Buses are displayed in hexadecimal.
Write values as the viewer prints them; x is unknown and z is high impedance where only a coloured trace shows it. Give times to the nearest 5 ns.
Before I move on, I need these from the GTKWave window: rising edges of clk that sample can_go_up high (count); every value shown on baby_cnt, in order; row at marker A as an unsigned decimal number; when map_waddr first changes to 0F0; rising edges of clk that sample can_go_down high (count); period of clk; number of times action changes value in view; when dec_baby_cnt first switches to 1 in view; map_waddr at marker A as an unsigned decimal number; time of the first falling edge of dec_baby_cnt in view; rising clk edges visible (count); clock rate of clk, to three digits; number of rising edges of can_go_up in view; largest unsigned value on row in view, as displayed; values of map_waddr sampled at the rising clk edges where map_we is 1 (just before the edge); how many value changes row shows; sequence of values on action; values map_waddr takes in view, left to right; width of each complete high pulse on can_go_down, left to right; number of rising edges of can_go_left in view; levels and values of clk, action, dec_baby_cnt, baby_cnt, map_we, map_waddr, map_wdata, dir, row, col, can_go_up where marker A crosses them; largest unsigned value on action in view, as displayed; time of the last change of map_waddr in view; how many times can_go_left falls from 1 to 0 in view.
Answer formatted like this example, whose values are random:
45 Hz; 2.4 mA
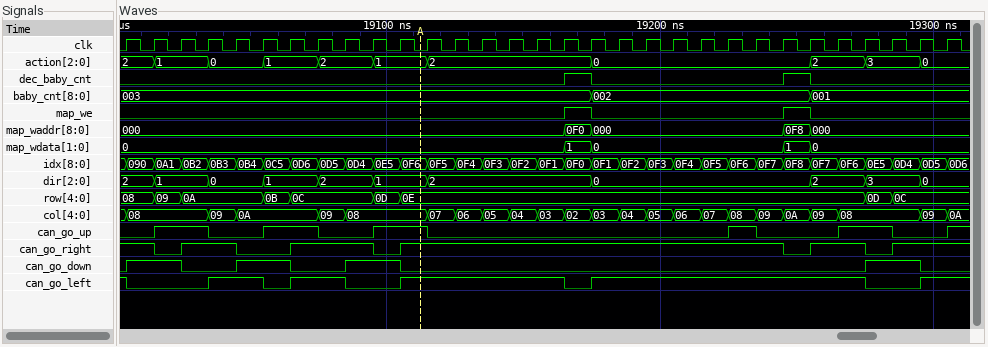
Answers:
9; 003, 002, 001; 14; 19165 ns; 8; 10 ns; 10; 19165 ns; 0; 19175 ns; 31; 100 MHz; 6; 0E; 0F0, 0F8; 8; 2, 1, 0, 1, 2, 1, 2, 0, 2, 3, 0; 000, 0F0, 000, 0F8, 000; 20 ns, 20 ns, 20 ns, 20 ns; 5; clk=0, action=1, dec_baby_cnt=0, baby_cnt=003, map_we=0, map_waddr=000, map_wdata=0, dir=1, row=0E, col=08, can_go_up=1; 3; 19255 ns; 5
